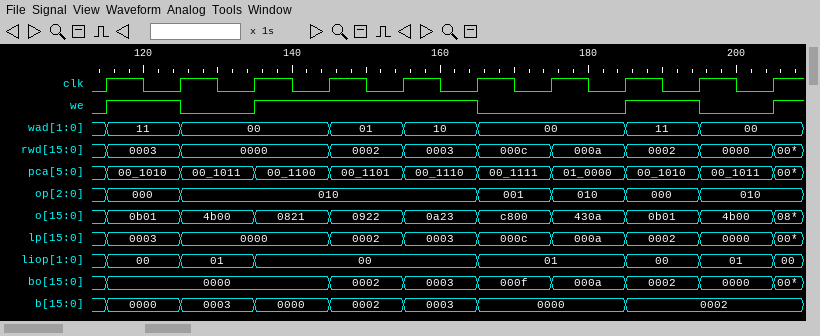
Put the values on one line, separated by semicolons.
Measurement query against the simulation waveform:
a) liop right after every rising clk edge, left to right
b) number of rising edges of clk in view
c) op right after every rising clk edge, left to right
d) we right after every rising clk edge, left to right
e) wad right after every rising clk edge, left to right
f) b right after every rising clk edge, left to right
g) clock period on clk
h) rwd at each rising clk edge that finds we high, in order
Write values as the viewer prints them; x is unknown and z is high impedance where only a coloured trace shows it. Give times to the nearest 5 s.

00, 01, 00, 00, 00, 01, 01, 00, 01, 00; 10; 000, 010, 010, 010, 010, 001, 010, 000, 010, 010; 1 0 1 1 1 0 0 1 0 1; 11, 00, 00, 01, 10, 00, 00, 11, 00, 00; 0000, 0003, 0000, 0002, 0003, 0000, 0000, 0002, 0002, 0002; 10 s; 0003, 0000, 0002, 0003, 0002
